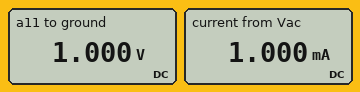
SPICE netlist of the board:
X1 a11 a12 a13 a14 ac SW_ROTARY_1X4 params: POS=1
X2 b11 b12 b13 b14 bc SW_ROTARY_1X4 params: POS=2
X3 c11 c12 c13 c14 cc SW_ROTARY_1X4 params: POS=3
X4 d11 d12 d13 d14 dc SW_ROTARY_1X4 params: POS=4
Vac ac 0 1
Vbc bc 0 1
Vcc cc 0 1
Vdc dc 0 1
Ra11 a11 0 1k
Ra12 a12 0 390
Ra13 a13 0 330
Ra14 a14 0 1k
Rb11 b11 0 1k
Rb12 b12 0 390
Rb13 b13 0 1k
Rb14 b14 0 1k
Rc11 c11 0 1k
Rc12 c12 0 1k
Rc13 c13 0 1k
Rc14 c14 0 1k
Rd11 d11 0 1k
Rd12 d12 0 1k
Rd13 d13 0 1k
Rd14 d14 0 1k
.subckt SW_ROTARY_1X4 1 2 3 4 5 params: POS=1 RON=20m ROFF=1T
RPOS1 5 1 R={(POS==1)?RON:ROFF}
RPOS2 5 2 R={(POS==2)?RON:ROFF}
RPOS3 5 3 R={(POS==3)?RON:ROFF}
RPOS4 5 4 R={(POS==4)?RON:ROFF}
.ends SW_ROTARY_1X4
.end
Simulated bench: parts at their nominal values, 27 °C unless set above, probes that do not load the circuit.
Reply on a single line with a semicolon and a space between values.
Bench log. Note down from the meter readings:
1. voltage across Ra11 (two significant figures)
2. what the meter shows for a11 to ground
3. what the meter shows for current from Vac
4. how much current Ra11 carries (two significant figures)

1.0 V; 1.000 V; 1.000 mA; 1.0 mA
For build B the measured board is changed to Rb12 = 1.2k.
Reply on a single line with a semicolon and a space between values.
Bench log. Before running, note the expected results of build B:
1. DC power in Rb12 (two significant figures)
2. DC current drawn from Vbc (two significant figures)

830 µW; 830 µA
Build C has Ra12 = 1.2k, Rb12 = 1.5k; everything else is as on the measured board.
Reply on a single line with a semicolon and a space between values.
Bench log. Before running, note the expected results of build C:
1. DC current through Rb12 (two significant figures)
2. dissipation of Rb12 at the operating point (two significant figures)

670 µA; 670 µW
